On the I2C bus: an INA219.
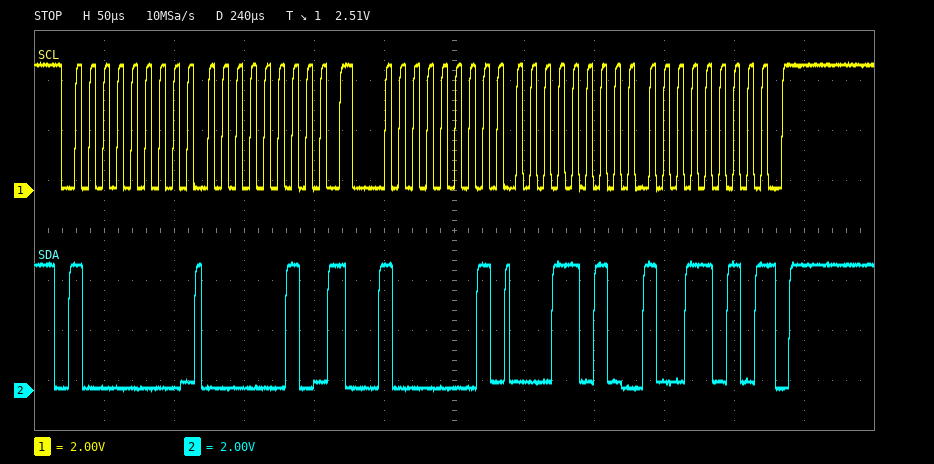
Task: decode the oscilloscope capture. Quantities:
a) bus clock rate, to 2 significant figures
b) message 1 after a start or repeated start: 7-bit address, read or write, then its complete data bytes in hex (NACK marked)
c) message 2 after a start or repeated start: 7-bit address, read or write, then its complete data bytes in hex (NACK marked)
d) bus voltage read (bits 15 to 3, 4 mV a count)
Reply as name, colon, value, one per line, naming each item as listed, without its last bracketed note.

bus clock rate, to 2 significant figures: 100 kHz
message 1 after a start or repeated start: 7-bit address, read or write, then its complete data bytes in hex: 0x40 write: 02
message 2 after a start or repeated start: 7-bit address, read or write, then its complete data bytes in hex: 0x40 read: 1A 9A NACK
bus voltage read: 3.404 V
